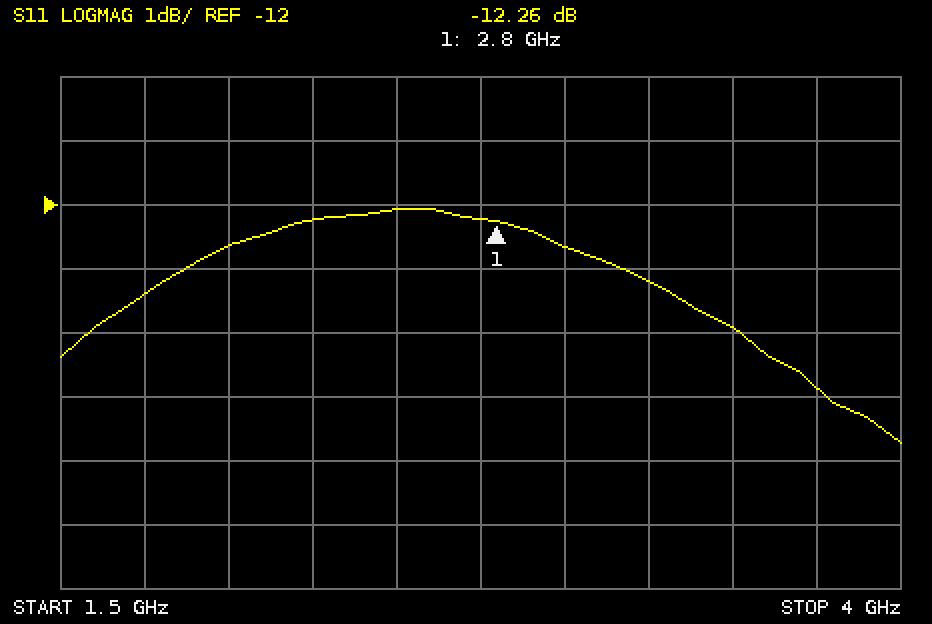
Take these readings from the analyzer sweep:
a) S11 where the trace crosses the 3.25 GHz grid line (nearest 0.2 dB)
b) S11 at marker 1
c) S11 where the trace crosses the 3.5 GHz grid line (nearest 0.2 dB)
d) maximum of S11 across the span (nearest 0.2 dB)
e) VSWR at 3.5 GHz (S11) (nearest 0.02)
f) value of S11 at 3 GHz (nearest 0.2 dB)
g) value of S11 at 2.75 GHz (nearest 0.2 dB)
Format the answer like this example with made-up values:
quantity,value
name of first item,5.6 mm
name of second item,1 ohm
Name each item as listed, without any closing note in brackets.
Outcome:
quantity,value
S11 where the trace crosses the 3.25 GHz grid line,-13.2 dB
S11 at marker 1,-12.26 dB
S11 where the trace crosses the 3.5 GHz grid line,-14.0 dB
maximum of S11 across the span,-12.0 dB
VSWR at 3.5 GHz (S11),1.50
value of S11 at 3 GHz,-12.6 dB
value of S11 at 2.75 GHz,-12.2 dB
